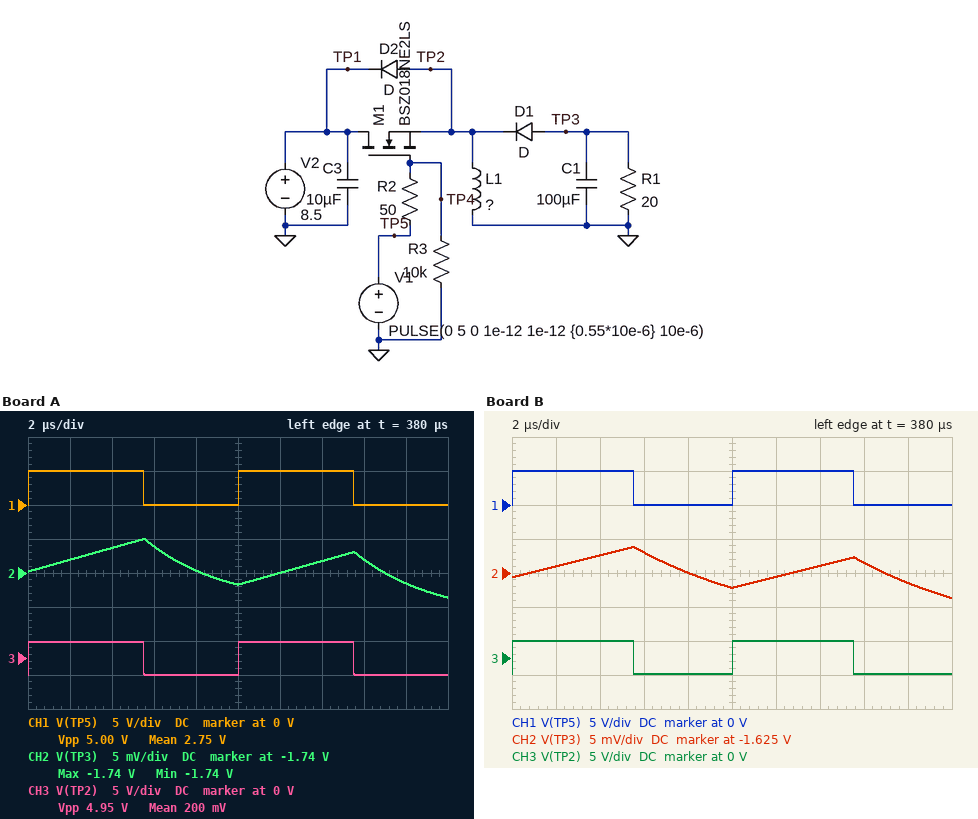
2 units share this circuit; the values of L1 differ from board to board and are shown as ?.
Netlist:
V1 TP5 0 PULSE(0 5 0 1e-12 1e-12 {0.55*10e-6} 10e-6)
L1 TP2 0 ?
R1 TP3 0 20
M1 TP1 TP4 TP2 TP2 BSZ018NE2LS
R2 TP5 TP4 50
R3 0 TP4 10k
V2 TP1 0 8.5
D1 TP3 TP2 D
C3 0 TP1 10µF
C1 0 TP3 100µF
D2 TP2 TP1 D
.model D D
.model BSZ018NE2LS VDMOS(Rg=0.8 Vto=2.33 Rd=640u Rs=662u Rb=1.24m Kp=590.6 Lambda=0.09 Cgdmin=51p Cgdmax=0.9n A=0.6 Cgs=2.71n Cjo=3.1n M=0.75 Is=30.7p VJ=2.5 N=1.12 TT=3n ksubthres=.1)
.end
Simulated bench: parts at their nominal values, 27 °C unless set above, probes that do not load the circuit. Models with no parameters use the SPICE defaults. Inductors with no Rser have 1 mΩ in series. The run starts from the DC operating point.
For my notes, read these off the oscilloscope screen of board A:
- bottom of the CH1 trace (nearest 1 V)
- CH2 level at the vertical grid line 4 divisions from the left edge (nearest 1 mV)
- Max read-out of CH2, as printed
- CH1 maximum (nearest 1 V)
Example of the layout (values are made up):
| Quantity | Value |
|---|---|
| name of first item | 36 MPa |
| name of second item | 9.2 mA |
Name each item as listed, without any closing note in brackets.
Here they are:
| Quantity | Value |
|---|---|
| bottom of the CH1 trace | 0 V |
| CH2 level at the vertical grid line 4 divisions from the left edge | -1.740 V |
| Max read-out of CH2, as printed | -1.74 V |
| CH1 maximum | 5 V |
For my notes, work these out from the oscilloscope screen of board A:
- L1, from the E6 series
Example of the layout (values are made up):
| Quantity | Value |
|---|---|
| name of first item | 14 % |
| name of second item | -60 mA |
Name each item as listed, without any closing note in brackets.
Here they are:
| Quantity | Value |
|---|---|
| L1, from the E6 series | 4.7 µH |
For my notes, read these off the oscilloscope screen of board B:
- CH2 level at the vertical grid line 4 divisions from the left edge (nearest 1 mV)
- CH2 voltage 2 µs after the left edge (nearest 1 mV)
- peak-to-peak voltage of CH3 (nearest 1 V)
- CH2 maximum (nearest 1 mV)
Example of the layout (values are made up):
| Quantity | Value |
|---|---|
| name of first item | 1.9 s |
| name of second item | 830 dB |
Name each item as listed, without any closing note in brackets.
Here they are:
| Quantity | Value |
|---|---|
| CH2 level at the vertical grid line 4 divisions from the left edge | -1.625 V |
| CH2 voltage 2 µs after the left edge | -1.624 V |
| peak-to-peak voltage of CH3 | 5 V |
| CH2 maximum | -1.621 V |
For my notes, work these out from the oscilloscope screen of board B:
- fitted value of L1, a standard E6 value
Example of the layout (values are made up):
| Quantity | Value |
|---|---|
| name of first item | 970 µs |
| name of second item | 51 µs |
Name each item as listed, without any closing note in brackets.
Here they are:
| Quantity | Value |
|---|---|
| fitted value of L1, a standard E6 value | 22 µH |
